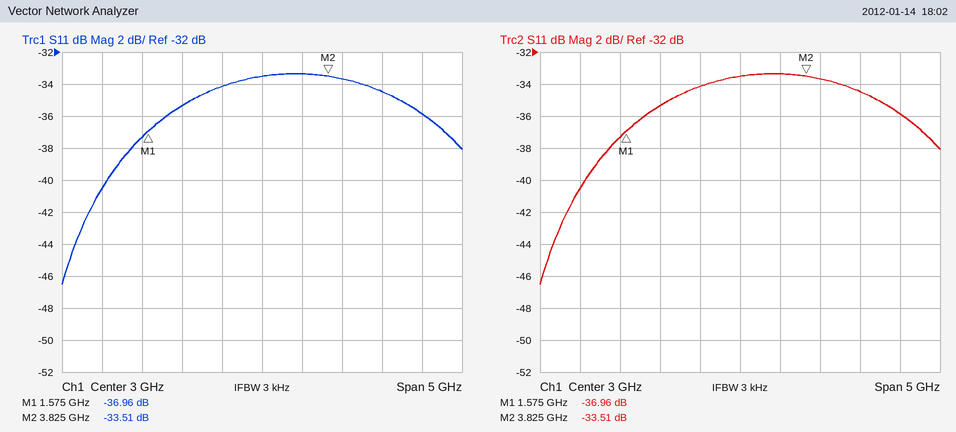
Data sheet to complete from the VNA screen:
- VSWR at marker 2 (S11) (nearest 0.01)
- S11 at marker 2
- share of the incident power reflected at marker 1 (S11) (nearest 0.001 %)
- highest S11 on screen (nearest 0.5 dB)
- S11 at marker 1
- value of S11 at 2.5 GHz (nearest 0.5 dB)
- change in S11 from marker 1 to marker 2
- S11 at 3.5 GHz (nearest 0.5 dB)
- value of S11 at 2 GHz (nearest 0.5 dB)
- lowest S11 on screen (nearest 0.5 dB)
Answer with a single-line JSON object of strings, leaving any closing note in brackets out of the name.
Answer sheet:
{"VSWR at marker 2 (S11)": "1.04", "S11 at marker 2": "-33.51 dB", "share of the incident power reflected at marker 1 (S11)": "0.020 %", "highest S11 on screen": "-33.5 dB", "S11 at marker 1": "-36.96 dB", "value of S11 at 2.5 GHz": "-34.0 dB", "change in S11 from marker 1 to marker 2": "3.45 dB", "S11 at 3.5 GHz": "-33.5 dB", "value of S11 at 2 GHz": "-35.5 dB", "lowest S11 on screen": "-46.5 dB"}
